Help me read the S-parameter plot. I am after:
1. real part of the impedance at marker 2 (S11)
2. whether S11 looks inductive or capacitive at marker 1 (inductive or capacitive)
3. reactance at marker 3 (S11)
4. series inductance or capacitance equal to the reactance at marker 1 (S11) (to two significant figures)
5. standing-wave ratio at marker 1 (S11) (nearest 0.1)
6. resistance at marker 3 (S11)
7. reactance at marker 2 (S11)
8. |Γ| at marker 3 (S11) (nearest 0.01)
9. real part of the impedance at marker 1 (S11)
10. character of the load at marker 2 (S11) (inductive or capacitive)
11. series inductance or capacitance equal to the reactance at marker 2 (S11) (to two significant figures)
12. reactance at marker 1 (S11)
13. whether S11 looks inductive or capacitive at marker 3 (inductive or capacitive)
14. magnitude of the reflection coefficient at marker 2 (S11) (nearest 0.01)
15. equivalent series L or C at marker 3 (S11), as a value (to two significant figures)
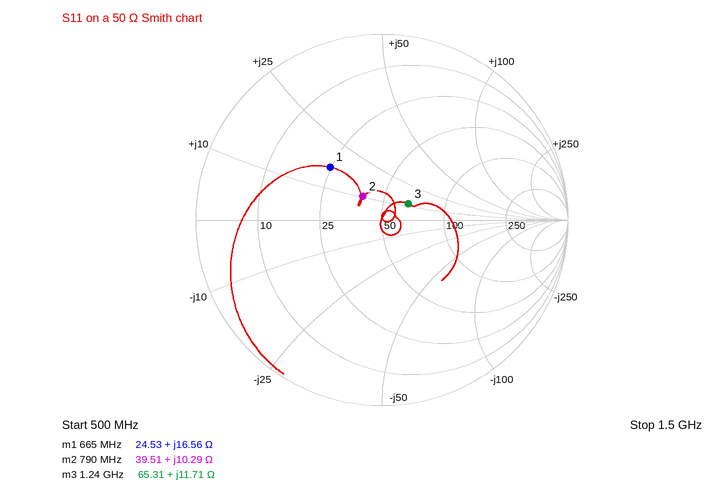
39.51 Ω
inductive
+11.71 Ω
4.0 nH
2.3
65.31 Ω
+10.29 Ω
0.17
24.53 Ω
inductive
2.1 nH
+16.56 Ω
inductive
0.16
1.5 nH
